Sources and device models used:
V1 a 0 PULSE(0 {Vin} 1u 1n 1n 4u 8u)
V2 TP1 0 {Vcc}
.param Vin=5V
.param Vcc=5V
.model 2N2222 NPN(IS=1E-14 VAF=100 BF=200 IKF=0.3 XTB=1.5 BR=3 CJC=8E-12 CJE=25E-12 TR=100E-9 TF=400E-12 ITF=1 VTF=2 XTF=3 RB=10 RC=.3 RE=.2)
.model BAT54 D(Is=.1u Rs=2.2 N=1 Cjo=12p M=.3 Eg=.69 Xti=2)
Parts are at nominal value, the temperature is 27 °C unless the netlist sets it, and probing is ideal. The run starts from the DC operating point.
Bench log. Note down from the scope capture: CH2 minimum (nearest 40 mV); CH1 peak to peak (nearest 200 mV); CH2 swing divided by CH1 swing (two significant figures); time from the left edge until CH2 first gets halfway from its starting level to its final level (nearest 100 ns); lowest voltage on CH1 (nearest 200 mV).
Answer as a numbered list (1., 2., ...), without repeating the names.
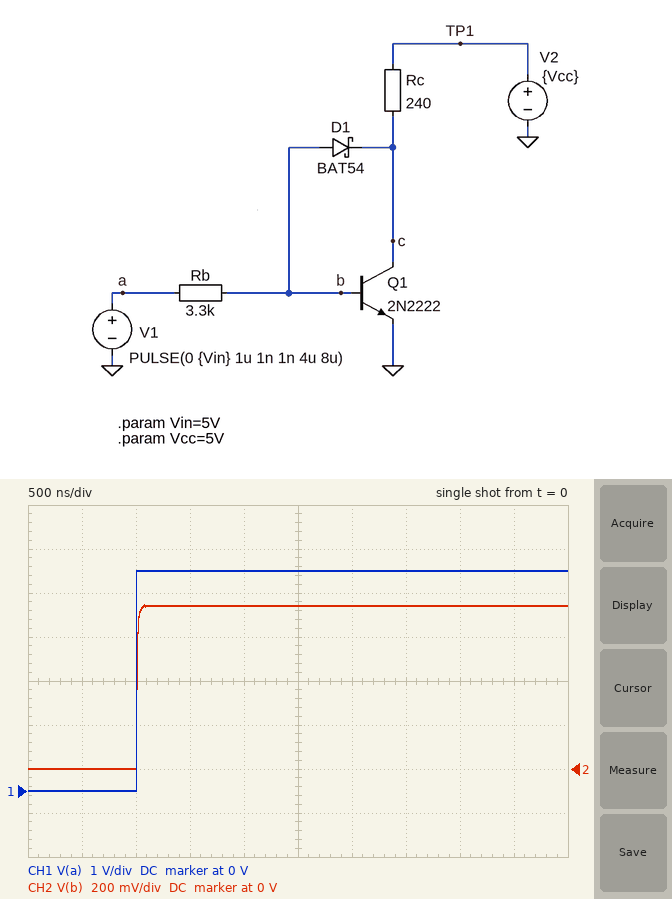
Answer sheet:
1. 0 V
2. 5.0 V
3. 0.15
4. 1.0 µs
5. 0 V
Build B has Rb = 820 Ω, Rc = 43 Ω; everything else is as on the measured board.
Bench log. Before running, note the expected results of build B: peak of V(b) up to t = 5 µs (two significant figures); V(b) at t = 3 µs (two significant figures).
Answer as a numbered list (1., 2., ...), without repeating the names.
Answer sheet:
1. 840 mV
2. 810 mV
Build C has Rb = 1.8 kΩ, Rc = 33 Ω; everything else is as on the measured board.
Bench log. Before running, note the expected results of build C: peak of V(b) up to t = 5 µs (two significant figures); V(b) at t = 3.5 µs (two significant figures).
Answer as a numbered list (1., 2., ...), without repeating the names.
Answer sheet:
1. 840 mV
2. 830 mV
